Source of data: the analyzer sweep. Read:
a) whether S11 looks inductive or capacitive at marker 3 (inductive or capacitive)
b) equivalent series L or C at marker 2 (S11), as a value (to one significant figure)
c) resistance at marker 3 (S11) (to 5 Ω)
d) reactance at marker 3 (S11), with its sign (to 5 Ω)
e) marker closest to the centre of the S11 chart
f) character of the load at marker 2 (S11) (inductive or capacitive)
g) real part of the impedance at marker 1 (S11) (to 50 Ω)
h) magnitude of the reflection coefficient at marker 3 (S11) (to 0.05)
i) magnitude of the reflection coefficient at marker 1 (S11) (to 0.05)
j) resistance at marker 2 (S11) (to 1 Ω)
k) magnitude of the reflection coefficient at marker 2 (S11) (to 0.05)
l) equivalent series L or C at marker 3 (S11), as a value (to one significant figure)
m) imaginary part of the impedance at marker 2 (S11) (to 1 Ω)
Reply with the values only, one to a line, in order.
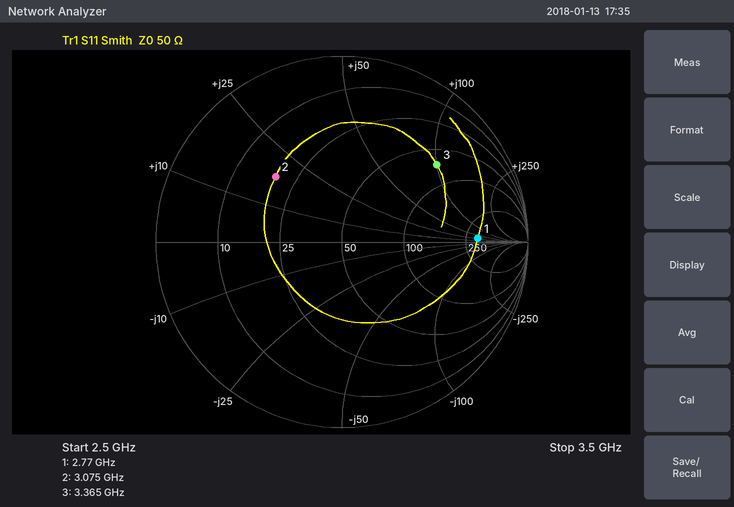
inductive
900 pH
70 Ω
+100 Ω
marker 2
inductive
300 Ω
0.65
0.75
19 Ω
0.50
5 nH
+18 Ω
